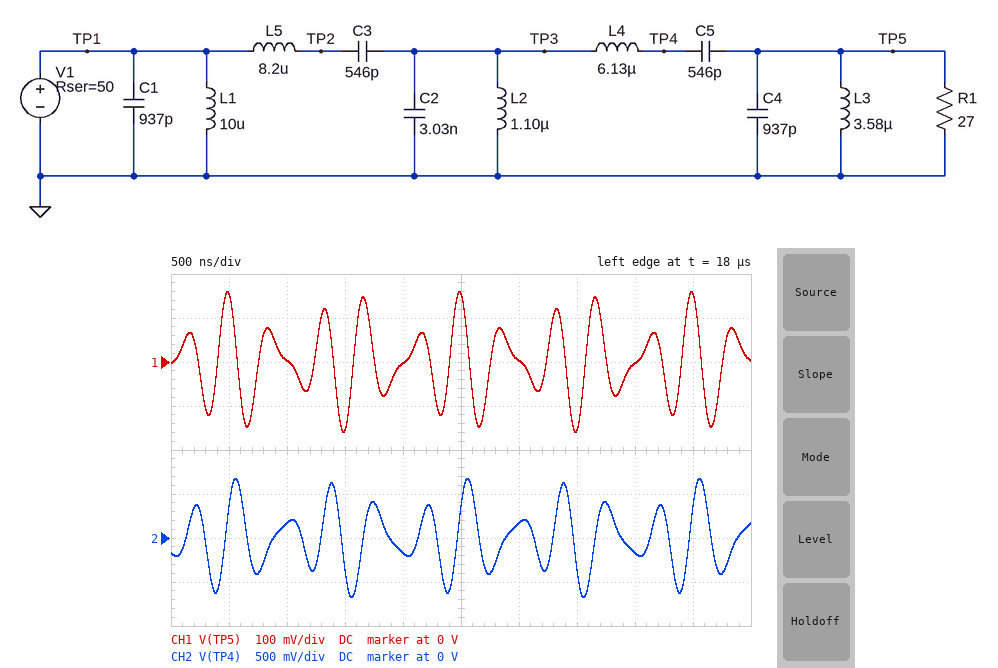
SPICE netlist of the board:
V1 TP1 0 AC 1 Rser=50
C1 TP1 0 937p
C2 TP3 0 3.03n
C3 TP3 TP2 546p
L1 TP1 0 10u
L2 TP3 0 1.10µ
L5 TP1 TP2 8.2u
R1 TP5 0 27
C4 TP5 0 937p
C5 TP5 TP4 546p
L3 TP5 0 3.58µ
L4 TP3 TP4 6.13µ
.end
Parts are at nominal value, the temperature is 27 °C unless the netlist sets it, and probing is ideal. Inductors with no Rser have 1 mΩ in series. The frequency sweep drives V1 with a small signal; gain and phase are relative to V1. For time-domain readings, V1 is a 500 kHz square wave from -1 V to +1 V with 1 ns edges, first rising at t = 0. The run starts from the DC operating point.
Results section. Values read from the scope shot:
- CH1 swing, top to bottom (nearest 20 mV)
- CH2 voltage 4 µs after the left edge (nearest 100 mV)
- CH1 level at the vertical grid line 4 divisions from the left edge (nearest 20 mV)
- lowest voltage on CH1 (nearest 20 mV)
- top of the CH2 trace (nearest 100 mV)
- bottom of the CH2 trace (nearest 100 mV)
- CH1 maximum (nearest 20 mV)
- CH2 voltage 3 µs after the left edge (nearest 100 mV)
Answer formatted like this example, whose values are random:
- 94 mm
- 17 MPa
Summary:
- 320 mV
- -200 mV
- 0 V
- -160 mV
- 700 mV
- -700 mV
- 160 mV
- 200 mV
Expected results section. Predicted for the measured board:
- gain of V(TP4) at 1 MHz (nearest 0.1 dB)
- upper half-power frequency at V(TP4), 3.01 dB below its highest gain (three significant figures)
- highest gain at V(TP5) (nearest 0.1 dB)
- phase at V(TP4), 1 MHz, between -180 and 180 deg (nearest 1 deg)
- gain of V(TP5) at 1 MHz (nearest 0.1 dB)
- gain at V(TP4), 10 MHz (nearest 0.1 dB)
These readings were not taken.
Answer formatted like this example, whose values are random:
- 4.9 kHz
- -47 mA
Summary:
- -28.0 dB
- 2.88 MHz
- -8.8 dB
- -165 deg
- -51.5 dB
- -65.9 dB
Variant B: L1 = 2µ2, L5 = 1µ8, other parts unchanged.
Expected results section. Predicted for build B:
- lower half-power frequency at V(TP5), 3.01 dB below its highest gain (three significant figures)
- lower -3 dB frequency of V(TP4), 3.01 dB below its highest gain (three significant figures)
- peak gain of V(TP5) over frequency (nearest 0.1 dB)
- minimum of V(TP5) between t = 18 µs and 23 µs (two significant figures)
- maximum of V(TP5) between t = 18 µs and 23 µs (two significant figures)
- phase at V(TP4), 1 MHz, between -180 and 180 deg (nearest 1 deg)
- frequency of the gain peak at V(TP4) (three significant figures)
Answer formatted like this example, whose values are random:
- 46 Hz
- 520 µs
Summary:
- 2.04 MHz
- 2.02 MHz
- -9.2 dB
- -110 mV
- 110 mV
- -108 deg
- 2.13 MHz
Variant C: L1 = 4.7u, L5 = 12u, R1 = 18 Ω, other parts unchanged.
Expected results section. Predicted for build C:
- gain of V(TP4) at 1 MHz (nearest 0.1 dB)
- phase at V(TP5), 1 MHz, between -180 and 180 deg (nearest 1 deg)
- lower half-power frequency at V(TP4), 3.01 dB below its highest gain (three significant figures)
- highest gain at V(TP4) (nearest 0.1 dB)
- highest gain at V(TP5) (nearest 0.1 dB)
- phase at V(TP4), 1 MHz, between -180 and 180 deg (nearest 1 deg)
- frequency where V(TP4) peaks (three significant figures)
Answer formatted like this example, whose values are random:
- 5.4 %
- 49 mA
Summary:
- -30.5 dB
- -9 deg
- 2.11 MHz
- 6.1 dB
- -10.7 dB
- -131 deg
- 2.33 MHz
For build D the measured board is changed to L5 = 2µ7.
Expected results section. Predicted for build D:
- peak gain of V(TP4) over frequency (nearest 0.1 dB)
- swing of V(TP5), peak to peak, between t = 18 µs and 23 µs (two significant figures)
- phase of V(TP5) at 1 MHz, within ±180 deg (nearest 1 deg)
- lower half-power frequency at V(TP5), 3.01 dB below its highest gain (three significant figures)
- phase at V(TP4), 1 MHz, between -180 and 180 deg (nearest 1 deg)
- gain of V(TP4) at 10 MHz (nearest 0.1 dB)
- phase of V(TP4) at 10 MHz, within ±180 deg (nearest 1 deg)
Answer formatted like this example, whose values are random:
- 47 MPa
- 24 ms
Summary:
- 4.1 dB
- 200 mV
- -30 deg
- 2.04 MHz
- -163 deg
- -54.1 dB
- -55 deg
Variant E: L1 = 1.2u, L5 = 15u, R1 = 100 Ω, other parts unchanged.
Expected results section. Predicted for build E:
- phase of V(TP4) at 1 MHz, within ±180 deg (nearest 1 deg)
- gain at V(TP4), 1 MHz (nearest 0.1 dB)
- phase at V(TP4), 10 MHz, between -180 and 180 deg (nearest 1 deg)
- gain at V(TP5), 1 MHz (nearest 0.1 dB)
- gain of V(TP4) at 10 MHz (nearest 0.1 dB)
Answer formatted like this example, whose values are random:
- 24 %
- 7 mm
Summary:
- -100 deg
- -41.6 dB
- -61 deg
- -62.2 dB
- -68.8 dB
